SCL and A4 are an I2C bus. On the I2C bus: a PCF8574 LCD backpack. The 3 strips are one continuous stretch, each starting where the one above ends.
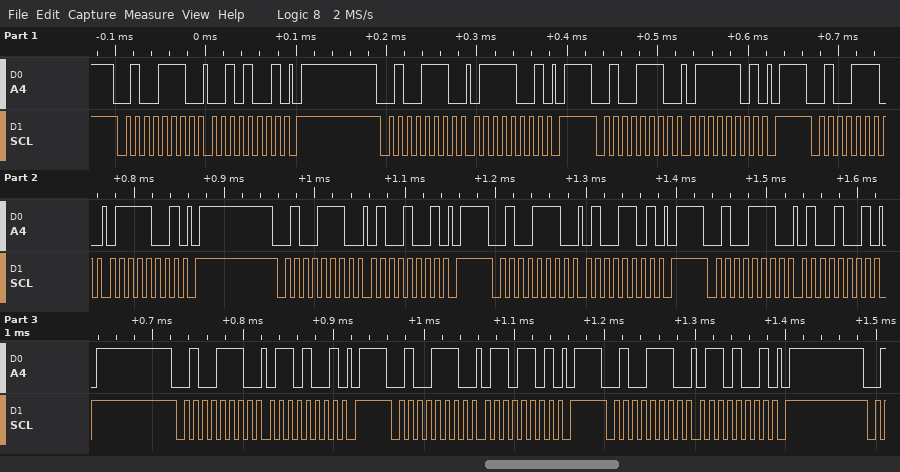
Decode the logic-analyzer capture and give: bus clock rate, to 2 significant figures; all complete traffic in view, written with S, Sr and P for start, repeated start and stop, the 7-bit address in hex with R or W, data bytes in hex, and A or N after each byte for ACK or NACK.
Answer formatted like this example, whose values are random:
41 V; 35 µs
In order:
100 kHz; S 27W A 29 A P S 27W A 79 A P S 27W A 7D A P S 27W A 79 A P S 27W A 49 A P S 27W A 4D A P S 27W A 49 A P S 27W A 69 A P S 27W A 6D A P S 27W A 69 A P
